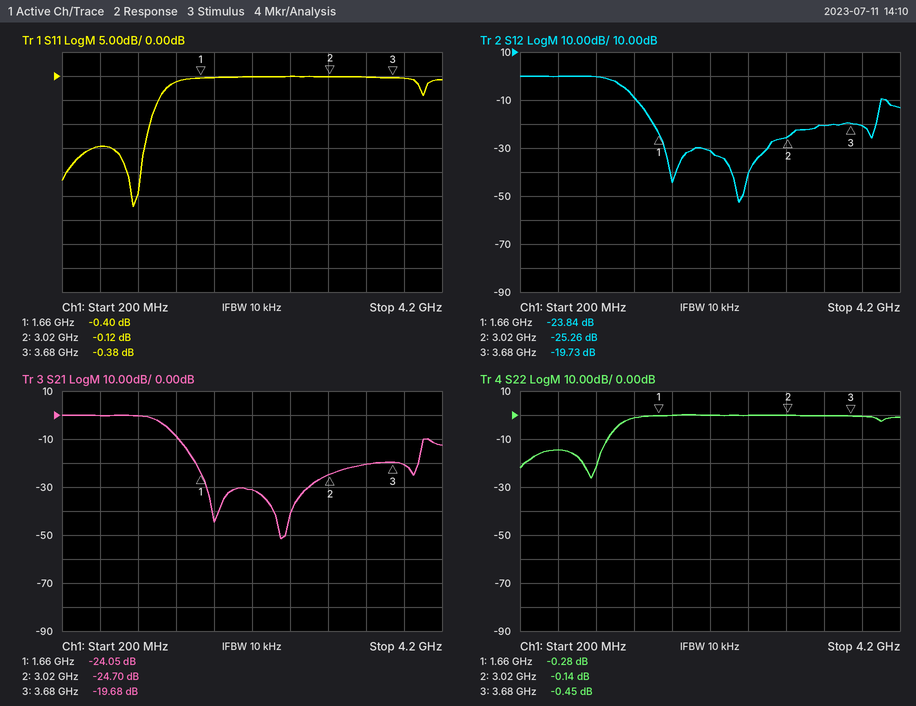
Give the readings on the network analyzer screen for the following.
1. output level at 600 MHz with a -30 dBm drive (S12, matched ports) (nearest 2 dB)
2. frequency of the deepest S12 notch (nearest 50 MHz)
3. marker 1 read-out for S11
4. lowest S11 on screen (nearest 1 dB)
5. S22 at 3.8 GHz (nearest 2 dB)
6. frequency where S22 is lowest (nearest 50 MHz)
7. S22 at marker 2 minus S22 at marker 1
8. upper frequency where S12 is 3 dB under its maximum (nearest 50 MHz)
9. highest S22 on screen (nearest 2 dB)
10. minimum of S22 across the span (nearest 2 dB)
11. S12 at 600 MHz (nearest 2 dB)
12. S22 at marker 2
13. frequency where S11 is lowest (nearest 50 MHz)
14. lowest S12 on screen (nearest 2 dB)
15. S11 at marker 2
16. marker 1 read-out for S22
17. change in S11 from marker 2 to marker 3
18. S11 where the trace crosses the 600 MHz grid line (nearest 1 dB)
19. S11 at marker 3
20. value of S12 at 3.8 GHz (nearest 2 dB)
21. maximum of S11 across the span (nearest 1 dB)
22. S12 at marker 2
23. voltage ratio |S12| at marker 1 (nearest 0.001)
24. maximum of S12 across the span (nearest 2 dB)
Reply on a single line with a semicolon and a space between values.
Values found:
-30 dBm; 2.50 GHz; -0.40 dB; -27 dB; 0 dB; 950 MHz; 0.14 dB; 1.25 GHz; 0 dB; -26 dB; 0 dB; -0.14 dB; 950 MHz; -52 dB; -0.12 dB; -0.28 dB; -0.26 dB; -15 dB; -0.38 dB; -20 dB; 0 dB; -25.26 dB; 0.064; 0 dB
